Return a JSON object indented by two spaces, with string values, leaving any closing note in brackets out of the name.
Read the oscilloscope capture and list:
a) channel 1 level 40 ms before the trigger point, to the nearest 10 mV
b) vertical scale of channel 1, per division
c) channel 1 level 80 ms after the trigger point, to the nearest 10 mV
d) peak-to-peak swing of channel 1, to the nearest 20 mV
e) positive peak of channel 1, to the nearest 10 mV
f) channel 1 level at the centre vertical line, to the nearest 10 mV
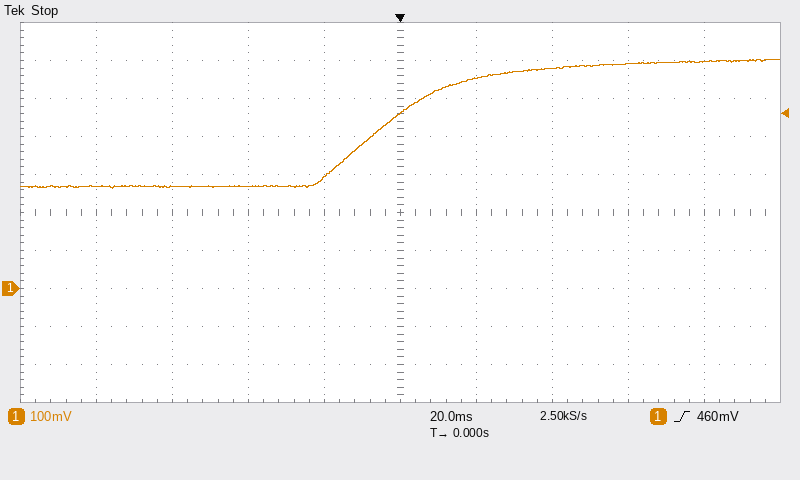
{
  "channel 1 level 40 ms before the trigger point, to the nearest 10 mV": "270 mV",
  "vertical scale of channel 1, per division": "100 mV",
  "channel 1 level 80 ms after the trigger point, to the nearest 10 mV": "600 mV",
  "peak-to-peak swing of channel 1, to the nearest 20 mV": "340 mV",
  "positive peak of channel 1, to the nearest 10 mV": "600 mV",
  "channel 1 level at the centre vertical line, to the nearest 10 mV": "460 mV"
}
